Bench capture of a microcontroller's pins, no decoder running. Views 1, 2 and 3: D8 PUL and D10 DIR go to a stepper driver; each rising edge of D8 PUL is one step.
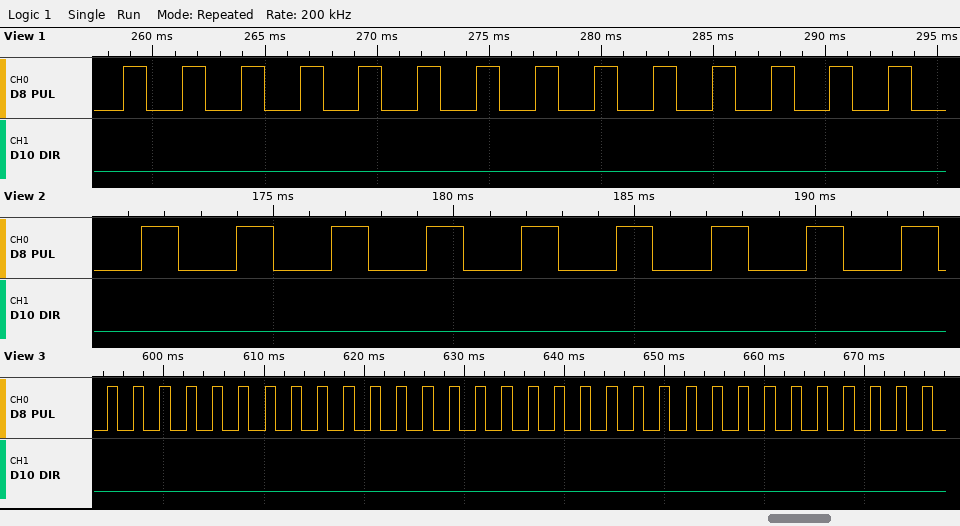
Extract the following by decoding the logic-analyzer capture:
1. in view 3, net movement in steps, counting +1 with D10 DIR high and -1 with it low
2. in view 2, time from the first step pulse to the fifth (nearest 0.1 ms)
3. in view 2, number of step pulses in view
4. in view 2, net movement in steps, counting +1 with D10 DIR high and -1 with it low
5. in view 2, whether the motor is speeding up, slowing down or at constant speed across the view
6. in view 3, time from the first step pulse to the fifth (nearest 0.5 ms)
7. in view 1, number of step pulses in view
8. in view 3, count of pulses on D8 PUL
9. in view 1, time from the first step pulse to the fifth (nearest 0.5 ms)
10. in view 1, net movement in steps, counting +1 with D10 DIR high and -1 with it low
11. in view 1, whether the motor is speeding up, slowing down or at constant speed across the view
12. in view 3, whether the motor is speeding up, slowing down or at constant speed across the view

-32
10.5 ms
9
-9
constant speed
10.5 ms
14
32
10.5 ms
-14
constant speed
constant speed
